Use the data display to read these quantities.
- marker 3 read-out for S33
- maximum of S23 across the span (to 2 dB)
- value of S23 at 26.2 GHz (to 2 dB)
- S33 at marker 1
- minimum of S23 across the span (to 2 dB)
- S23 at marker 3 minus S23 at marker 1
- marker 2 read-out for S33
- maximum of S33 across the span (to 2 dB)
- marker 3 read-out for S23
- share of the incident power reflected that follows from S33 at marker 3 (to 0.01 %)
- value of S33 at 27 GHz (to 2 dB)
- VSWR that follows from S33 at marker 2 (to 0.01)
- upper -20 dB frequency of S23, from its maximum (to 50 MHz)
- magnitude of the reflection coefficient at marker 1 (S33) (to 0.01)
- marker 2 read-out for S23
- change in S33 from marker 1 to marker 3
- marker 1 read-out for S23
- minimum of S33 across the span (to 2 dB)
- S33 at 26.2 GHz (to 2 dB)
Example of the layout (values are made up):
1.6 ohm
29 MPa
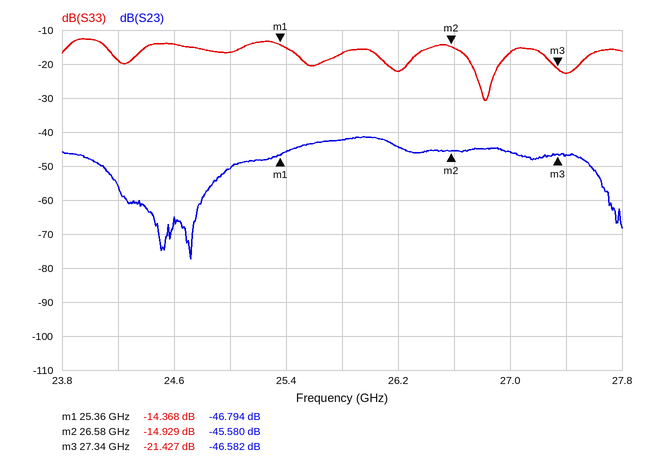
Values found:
-21.427 dB
-42 dB
-44 dB
-14.368 dB
-78 dB
0.212 dB
-14.929 dB
-12 dB
-46.582 dB
0.72 %
-16 dB
1.44
27.70 GHz
0.19
-45.580 dB
-7.059 dB
-46.794 dB
-30 dB
-22 dB
